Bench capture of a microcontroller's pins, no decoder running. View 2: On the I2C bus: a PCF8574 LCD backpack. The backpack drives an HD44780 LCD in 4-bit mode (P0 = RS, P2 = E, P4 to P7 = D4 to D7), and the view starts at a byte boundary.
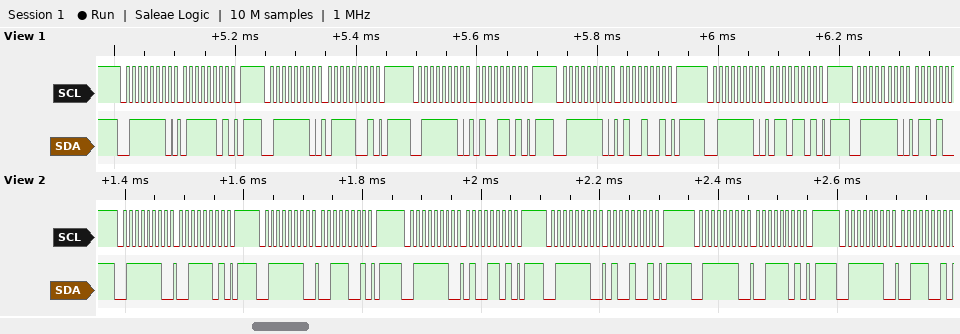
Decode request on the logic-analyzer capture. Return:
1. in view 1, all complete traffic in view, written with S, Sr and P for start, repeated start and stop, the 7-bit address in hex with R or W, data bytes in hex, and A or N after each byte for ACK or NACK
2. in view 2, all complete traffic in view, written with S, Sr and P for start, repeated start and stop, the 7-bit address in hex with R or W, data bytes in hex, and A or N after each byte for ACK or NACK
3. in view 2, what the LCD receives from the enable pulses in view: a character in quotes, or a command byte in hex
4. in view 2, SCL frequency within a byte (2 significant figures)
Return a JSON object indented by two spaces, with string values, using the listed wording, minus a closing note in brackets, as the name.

{
  "in view 1, all complete traffic in view, written with S, Sr and P for start, repeated start and stop, the 7-bit address in hex with R or W, data bytes in hex, and A or N after each byte for ACK or NACK": "S 3FW A 7D A P S 3FW A 79 A P S 3FW A 4D A P S 3FW A 49 A P S 3FW A 6D A P S 3FW A",
  "in view 2, all complete traffic in view, written with S, Sr and P for start, repeated start and stop, the 7-bit address in hex with R or W, data bytes in hex, and A or N after each byte for ACK or NACK": "S 3FW A 3D A P S 3FW A 39 A P S 3FW A 4D A P S 3FW A 49 A P S 3FW A 3D A P S 3FW A 39 A",
  "in view 2, what the LCD receives from the enable pulses in view: a character in quotes, or a command byte in hex": "'4'",
  "in view 2, SCL frequency within a byte": "100 kHz"
}
